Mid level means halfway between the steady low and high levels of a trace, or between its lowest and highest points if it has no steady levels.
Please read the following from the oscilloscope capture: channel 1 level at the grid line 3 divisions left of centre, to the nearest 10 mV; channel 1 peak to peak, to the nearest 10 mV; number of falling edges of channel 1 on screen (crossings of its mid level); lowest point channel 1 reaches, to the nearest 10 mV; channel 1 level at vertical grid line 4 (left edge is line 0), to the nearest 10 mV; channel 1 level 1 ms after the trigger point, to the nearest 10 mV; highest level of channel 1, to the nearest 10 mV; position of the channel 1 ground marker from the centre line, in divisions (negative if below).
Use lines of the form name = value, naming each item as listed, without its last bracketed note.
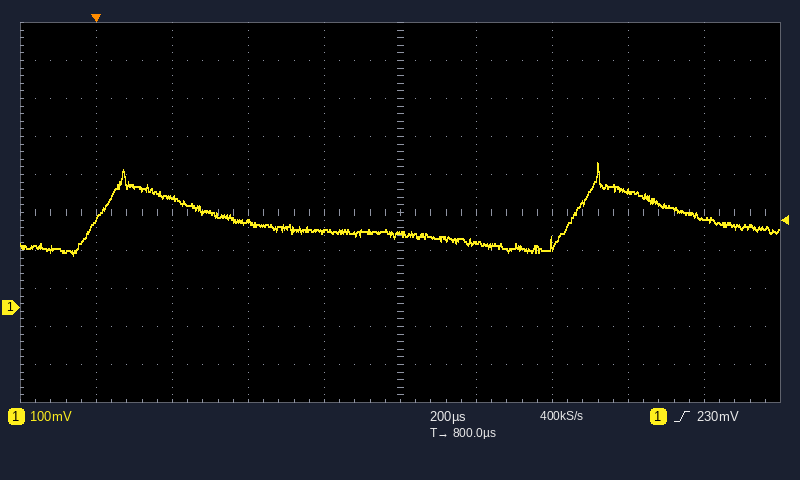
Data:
channel 1 level at the grid line 3 divisions left of centre, to the nearest 10 mV = 290 mV
channel 1 peak to peak, to the nearest 10 mV = 240 mV
number of falling edges of channel 1 on screen = 2
lowest point channel 1 reaches, to the nearest 10 mV = 140 mV
channel 1 level at vertical grid line 4 (left edge is line 0), to the nearest 10 mV = 200 mV
channel 1 level 1 ms after the trigger point, to the nearest 10 mV = 170 mV
highest level of channel 1, to the nearest 10 mV = 380 mV
position of the channel 1 ground marker from the centre line, in divisions = -2.5 div
